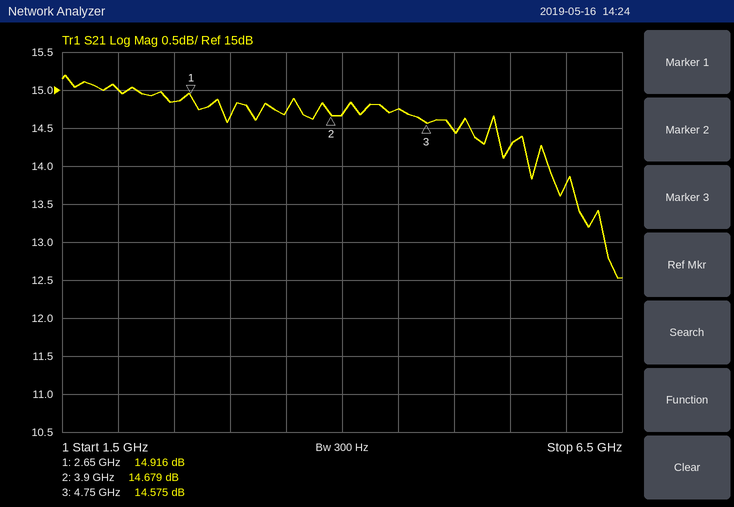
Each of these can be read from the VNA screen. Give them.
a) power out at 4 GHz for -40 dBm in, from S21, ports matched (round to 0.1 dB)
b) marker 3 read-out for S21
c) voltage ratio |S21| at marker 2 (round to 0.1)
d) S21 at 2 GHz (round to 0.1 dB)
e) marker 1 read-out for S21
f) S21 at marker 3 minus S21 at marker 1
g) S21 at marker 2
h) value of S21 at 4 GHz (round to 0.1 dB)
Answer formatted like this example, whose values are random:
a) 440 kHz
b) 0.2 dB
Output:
a) -25.3 dBm
b) 14.575 dB
c) 5.4
d) 15.0 dB
e) 14.916 dB
f) -0.341 dB
g) 14.679 dB
h) 14.7 dB
